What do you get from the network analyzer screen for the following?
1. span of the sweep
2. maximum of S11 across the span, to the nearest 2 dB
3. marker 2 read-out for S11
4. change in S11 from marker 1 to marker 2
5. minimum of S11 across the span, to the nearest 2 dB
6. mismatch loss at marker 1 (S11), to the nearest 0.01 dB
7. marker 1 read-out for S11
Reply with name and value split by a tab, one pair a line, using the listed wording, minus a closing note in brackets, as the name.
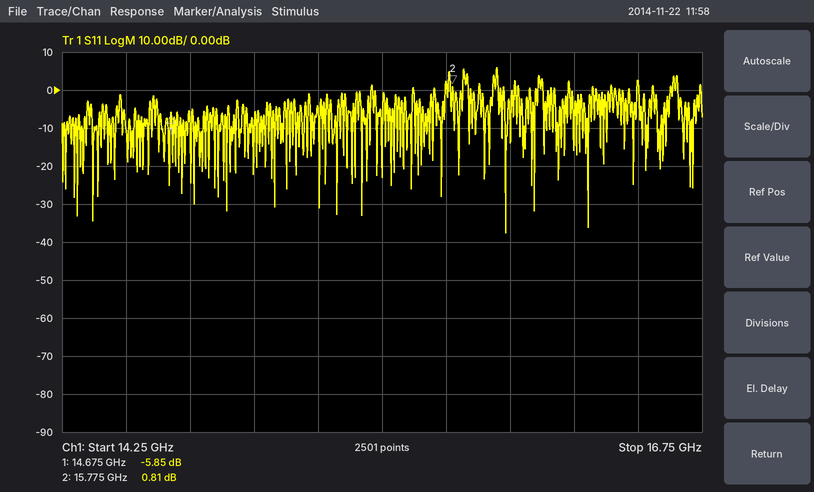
span of the sweep	2.5 GHz
maximum of S11 across the span, to the nearest 2 dB	6 dB
marker 2 read-out for S11	0.81 dB
change in S11 from marker 1 to marker 2	6.66 dB
minimum of S11 across the span, to the nearest 2 dB	-38 dB
mismatch loss at marker 1 (S11), to the nearest 0.01 dB	1.31 dB
marker 1 read-out for S11	-5.85 dB
